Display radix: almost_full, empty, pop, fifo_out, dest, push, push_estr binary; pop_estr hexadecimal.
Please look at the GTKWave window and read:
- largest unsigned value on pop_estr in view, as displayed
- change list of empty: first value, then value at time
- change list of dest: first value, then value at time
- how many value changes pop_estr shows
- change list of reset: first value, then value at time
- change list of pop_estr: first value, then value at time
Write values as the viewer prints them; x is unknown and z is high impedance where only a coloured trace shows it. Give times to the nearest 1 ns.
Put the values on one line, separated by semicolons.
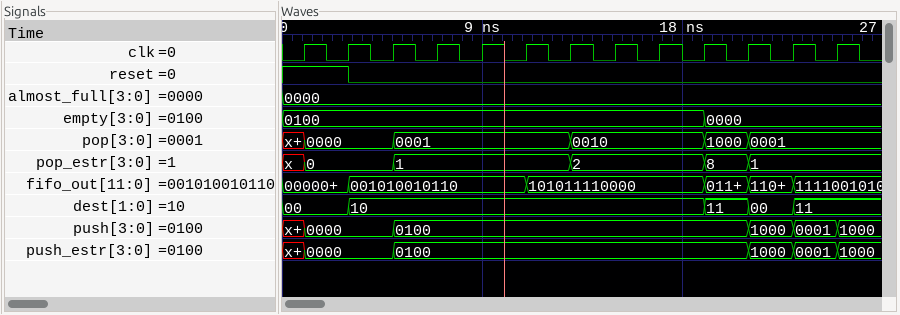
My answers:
8; 0100, 0000 at 19 ns; 00, 10 at 3 ns, 11 at 19 ns, 00 at 21 ns, 11 at 23 ns; 5; 1, 0 at 3 ns; x, 0 at 1 ns, 1 at 5 ns, 2 at 13 ns, 8 at 19 ns, 1 at 21 ns
